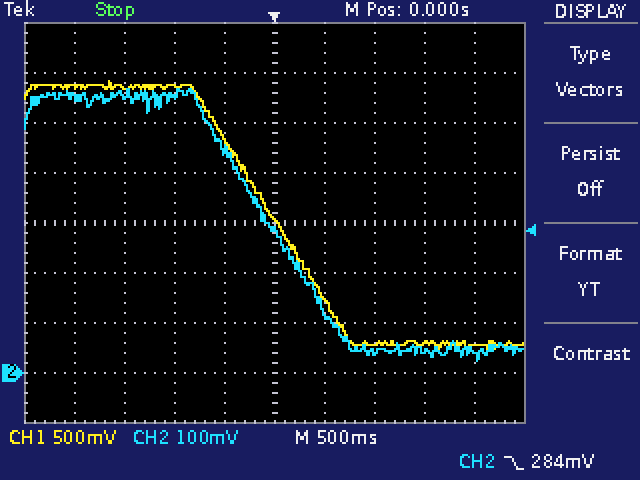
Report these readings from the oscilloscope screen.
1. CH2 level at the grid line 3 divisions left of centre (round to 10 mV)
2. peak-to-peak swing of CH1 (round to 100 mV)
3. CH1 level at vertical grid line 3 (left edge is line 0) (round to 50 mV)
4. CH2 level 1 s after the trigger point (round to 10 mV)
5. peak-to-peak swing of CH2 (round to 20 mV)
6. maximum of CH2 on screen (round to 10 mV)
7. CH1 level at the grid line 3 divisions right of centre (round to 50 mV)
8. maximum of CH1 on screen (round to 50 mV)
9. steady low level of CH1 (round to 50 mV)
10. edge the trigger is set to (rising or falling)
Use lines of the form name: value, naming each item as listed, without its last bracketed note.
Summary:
CH2 level at the grid line 3 divisions left of centre: 560 mV
peak-to-peak swing of CH1: 2.70 V
CH1 level at vertical grid line 3 (left edge is line 0): 2.85 V
CH2 level 1 s after the trigger point: 40 mV
peak-to-peak swing of CH2: 540 mV
maximum of CH2 on screen: 570 mV
CH1 level at the grid line 3 divisions right of centre: 300 mV
maximum of CH1 on screen: 2.90 V
steady low level of CH1: 300 mV
edge the trigger is set to: falling
